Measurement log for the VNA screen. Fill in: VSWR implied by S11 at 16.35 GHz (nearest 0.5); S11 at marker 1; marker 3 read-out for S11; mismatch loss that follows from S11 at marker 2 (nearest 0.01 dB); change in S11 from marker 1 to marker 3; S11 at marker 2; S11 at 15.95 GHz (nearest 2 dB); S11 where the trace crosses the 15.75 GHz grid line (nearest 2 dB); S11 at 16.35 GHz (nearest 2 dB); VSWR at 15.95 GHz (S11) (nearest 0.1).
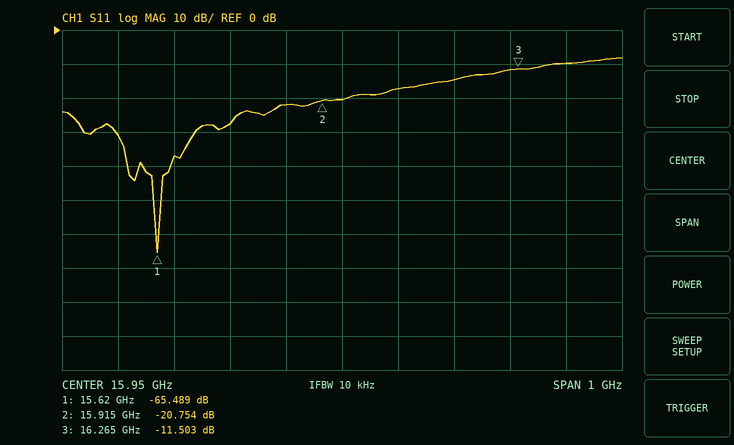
2.0
-65.489 dB
-11.503 dB
0.04 dB
53.986 dB
-20.754 dB
-20 dB
-28 dB
-10 dB
1.2
